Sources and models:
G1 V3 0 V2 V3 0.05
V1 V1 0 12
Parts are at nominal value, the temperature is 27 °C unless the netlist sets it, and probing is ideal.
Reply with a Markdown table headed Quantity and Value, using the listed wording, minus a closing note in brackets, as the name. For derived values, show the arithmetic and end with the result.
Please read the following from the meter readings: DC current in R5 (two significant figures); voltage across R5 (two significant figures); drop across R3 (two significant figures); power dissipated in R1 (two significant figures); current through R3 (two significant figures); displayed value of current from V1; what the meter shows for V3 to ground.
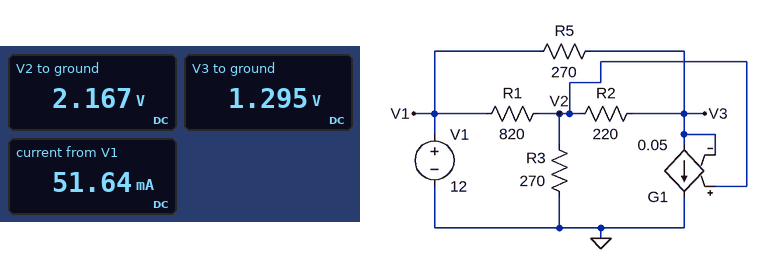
| Quantity | Value |
|---|---|
| DC current in R5 | (12 V - 1.295 V) / 270 Ω = 40 mA |
| voltage across R5 | 12 V - 1.295 V = 11 V |
| drop across R3 | 2.167 V = 2.2 V |
| power dissipated in R1 | (12 V - 2.167 V)^2 / 820 Ω = 120 mW |
| current through R3 | (2.167 V) / 270 Ω = 8.0 mA |
| displayed value of current from V1 | 51.64 mA |
| what the meter shows for V3 to ground | 1.295 V |
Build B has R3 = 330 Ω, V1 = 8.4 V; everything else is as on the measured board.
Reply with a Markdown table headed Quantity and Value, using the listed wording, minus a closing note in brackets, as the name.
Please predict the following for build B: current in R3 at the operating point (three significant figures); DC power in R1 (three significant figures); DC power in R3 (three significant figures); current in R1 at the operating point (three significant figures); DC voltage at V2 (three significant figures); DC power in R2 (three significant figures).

| Quantity | Value |
|---|---|
| current in R3 at the operating point | 5.40 mA |
| DC power in R1 | 53.4 mW |
| DC power in R3 | 9.63 mW |
| current in R1 at the operating point | 8.07 mA |
| DC voltage at V2 | 1.78 V |
| DC power in R2 | 1.57 mW |
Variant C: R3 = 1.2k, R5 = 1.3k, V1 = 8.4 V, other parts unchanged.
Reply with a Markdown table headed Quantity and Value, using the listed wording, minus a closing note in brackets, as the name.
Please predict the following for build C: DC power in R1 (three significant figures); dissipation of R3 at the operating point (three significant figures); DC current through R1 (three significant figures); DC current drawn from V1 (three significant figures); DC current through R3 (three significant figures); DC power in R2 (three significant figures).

| Quantity | Value |
|---|---|
| DC power in R1 | 15.3 mW |
| dissipation of R3 at the operating point | 19.6 mW |
| DC current through R1 | 4.32 mA |
| DC current drawn from V1 | 7.10 mA |
| DC current through R3 | 4.05 mA |
| DC power in R2 | 16.9 µW |
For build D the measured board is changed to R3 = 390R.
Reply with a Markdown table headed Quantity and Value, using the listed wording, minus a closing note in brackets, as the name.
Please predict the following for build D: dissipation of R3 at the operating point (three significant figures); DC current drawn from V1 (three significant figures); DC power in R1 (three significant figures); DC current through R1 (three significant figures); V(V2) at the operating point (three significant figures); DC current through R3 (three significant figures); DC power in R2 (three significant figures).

| Quantity | Value |
|---|---|
| dissipation of R3 at the operating point | 21.5 mW |
| DC current drawn from V1 | 47.8 mA |
| DC power in R1 | 101 mW |
| DC current through R1 | 11.1 mA |
| V(V2) at the operating point | 2.90 V |
| DC current through R3 | 7.43 mA |
| DC power in R2 | 2.96 mW |
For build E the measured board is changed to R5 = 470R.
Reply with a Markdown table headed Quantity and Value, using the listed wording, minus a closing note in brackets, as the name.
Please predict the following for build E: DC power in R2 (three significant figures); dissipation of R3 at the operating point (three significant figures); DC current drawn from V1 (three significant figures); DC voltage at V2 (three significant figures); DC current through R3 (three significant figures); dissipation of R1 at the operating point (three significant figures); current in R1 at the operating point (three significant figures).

| Quantity | Value |
|---|---|
| DC power in R2 | 980 µW |
| dissipation of R3 at the operating point | 24.0 mW |
| DC current drawn from V1 | 32.6 mA |
| DC voltage at V2 | 2.54 V |
| DC current through R3 | 9.42 mA |
| dissipation of R1 at the operating point | 109 mW |
| current in R1 at the operating point | 11.5 mA |
